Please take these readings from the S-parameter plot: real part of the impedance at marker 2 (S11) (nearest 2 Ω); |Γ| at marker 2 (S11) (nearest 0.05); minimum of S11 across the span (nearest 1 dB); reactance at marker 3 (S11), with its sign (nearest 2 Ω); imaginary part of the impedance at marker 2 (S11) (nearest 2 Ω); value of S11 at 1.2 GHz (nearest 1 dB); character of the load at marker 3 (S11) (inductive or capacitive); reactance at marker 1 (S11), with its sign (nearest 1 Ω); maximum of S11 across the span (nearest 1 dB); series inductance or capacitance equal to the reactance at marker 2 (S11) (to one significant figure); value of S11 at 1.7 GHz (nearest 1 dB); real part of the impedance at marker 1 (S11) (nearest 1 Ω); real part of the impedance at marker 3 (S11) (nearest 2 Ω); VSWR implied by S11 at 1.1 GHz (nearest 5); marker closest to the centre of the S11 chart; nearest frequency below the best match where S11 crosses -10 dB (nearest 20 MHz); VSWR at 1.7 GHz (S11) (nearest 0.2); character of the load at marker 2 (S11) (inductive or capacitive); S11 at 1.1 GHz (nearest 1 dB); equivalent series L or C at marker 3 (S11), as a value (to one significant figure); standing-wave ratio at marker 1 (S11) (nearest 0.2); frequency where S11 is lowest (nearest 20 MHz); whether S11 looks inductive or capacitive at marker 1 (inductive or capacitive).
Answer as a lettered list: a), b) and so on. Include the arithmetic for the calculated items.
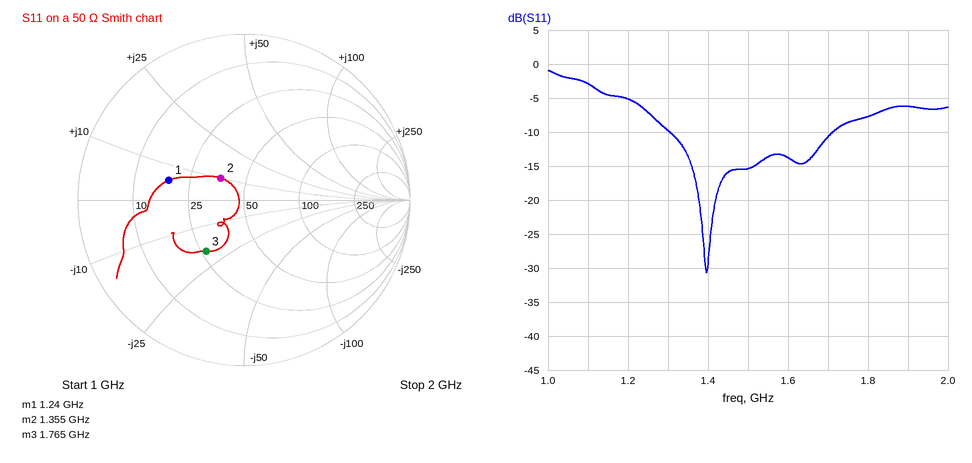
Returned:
a) 36 Ω
b) 0.20
c) -31 dB
d) -20 Ω
e) +10 Ω
f) -5 dB
g) capacitive
h) +6 Ω
i) -1 dB
j) L = 10 Ω/(2π × 1.355 GHz) ≈ 1 nH
k) -11 dB
l) 18 Ω
m) 26 Ω
n) |Γ| = 10^(-3/20) = 0.7079; VSWR = (1 + 0.7079)/(1 − 0.7079) ≈ 5.85, so 5 to the nearest 5
o) marker 2
p) 1.30 GHz
q) |Γ| = 10^(-11/20) = 0.2818; VSWR = (1 + 0.2818)/(1 − 0.2818) ≈ 1.8
r) inductive
s) -3 dB
t) C = 1/(2π × 1.765 GHz × 20 Ω) ≈ 5 pF
u) 2.8
v) 1.40 GHz
w) inductive
